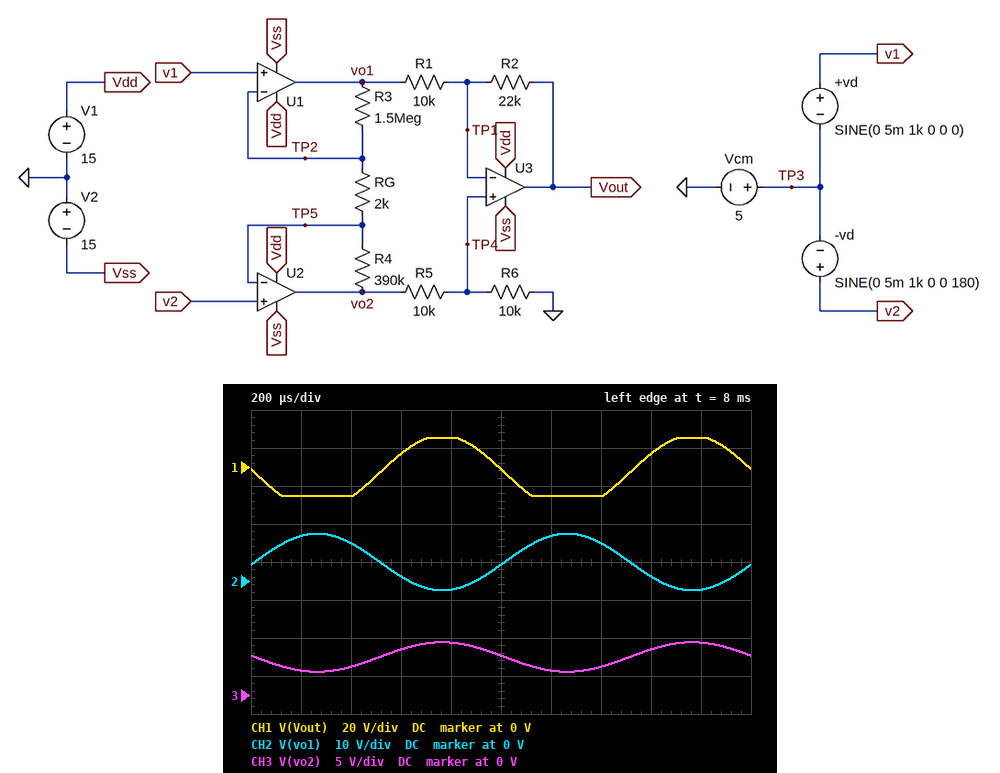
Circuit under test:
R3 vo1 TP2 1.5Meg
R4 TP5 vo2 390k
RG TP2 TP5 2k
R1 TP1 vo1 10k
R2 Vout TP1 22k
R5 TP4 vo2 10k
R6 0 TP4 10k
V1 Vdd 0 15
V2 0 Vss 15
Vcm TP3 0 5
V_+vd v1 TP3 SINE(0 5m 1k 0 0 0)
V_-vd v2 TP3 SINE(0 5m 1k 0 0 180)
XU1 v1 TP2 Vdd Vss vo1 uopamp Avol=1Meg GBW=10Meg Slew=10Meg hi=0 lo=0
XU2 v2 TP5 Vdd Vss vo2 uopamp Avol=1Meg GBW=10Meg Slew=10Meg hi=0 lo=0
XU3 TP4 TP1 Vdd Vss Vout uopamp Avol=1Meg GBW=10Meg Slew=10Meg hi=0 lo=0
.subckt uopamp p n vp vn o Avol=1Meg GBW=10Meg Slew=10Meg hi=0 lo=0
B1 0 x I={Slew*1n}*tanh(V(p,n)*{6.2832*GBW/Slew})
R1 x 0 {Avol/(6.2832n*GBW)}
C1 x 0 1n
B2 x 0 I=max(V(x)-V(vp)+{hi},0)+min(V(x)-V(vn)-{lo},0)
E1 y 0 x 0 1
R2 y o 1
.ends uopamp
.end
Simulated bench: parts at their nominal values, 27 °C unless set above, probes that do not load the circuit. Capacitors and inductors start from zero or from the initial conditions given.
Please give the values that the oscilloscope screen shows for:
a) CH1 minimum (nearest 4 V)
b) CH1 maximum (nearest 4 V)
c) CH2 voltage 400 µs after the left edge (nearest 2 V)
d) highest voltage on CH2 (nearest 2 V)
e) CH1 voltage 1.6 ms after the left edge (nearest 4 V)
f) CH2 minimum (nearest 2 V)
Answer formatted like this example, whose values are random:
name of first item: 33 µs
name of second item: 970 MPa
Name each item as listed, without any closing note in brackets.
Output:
CH1 minimum: -16 V
CH1 maximum: 16 V
CH2 voltage 400 µs after the left edge: 10 V
highest voltage on CH2: 12 V
CH1 voltage 1.6 ms after the left edge: 8 V
CH2 minimum: -2 V
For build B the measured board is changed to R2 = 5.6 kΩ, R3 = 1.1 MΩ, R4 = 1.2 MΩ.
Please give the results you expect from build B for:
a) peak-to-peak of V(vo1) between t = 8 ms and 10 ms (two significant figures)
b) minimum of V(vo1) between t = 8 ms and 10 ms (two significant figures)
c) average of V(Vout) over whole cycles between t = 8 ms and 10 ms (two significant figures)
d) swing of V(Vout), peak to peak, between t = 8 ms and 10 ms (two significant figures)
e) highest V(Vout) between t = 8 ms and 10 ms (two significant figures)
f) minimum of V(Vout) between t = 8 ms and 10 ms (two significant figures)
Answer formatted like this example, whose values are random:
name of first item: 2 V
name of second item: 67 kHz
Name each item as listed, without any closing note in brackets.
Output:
peak-to-peak of V(vo1) between t = 8 ms and 10 ms: 11 V
minimum of V(vo1) between t = 8 ms and 10 ms: -460 mV
average of V(Vout) over whole cycles between t = 8 ms and 10 ms: 1.1 V
swing of V(Vout), peak to peak, between t = 8 ms and 10 ms: 15 V
highest V(Vout) between t = 8 ms and 10 ms: 8.8 V
minimum of V(Vout) between t = 8 ms and 10 ms: -6.6 V
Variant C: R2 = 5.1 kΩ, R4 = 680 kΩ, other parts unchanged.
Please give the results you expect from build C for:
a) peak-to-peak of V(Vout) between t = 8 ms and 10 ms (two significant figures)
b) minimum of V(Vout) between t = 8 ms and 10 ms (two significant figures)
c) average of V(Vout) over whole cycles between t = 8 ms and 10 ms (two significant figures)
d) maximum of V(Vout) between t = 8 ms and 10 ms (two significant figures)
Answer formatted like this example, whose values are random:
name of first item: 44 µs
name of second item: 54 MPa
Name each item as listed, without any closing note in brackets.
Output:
peak-to-peak of V(Vout) between t = 8 ms and 10 ms: 13 V
minimum of V(Vout) between t = 8 ms and 10 ms: -5.1 V
average of V(Vout) over whole cycles between t = 8 ms and 10 ms: 1.2 V
maximum of V(Vout) between t = 8 ms and 10 ms: 7.6 V
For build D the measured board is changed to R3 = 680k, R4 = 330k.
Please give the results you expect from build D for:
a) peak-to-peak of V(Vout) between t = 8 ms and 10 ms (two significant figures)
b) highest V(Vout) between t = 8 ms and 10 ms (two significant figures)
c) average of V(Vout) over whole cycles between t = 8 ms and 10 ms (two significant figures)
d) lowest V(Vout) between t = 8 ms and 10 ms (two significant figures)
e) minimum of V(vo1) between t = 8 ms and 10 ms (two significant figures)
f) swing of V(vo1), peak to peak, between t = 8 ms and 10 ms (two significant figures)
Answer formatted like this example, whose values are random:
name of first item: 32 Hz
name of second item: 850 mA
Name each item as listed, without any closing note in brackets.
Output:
peak-to-peak of V(Vout) between t = 8 ms and 10 ms: 20 V
highest V(Vout) between t = 8 ms and 10 ms: 7.1 V
average of V(Vout) over whole cycles between t = 8 ms and 10 ms: -3.0 V
lowest V(Vout) between t = 8 ms and 10 ms: -13 V
minimum of V(vo1) between t = 8 ms and 10 ms: 1.6 V
swing of V(vo1), peak to peak, between t = 8 ms and 10 ms: 6.8 V
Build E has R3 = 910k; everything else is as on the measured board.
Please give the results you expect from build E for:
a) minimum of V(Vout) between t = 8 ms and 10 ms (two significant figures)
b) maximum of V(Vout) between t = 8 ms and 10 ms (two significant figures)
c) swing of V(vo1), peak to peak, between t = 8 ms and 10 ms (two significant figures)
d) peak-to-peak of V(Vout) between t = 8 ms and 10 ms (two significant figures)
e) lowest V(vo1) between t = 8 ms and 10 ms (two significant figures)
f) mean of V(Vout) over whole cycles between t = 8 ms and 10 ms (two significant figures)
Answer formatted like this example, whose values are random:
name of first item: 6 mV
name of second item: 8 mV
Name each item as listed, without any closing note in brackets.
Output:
minimum of V(Vout) between t = 8 ms and 10 ms: -15 V
maximum of V(Vout) between t = 8 ms and 10 ms: 10 V
swing of V(vo1), peak to peak, between t = 8 ms and 10 ms: 9.1 V
peak-to-peak of V(Vout) between t = 8 ms and 10 ms: 25 V
lowest V(vo1) between t = 8 ms and 10 ms: 460 mV
mean of V(Vout) over whole cycles between t = 8 ms and 10 ms: -2.9 V
